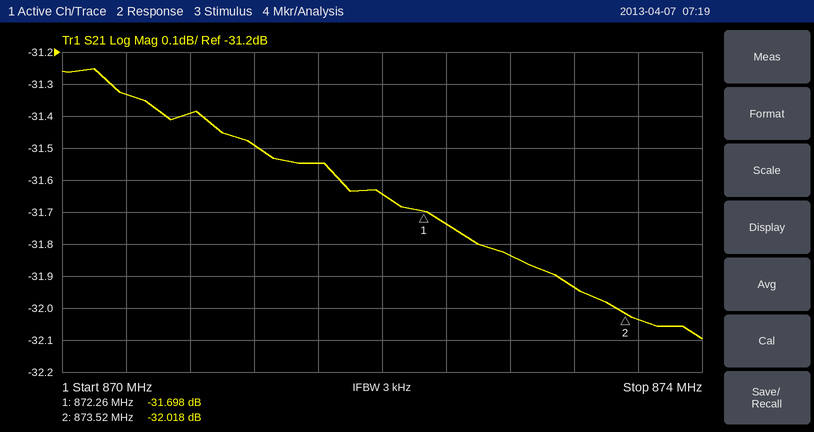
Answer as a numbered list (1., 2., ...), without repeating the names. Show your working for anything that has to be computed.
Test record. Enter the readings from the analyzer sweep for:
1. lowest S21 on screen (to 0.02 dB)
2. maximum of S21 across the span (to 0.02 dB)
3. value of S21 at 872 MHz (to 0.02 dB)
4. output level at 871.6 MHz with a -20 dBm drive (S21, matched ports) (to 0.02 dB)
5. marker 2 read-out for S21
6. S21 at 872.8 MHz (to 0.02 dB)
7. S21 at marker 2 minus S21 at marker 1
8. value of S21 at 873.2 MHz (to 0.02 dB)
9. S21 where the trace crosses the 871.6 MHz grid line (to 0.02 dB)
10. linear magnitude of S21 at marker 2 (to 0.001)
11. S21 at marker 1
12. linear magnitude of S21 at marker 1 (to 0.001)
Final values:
1. -32.10 dB
2. -31.26 dB
3. -31.64 dB
4. -20 dBm + (-31.54 dB) = -51.54 dBm
5. -32.018 dB
6. -31.84 dB
7. -32.018 − (-31.698) = -0.320 dB
8. -31.94 dB
9. -31.54 dB
10. 10^(-32.018/20) ≈ 0.025
11. -31.698 dB
12. 10^(-31.698/20) ≈ 0.026
